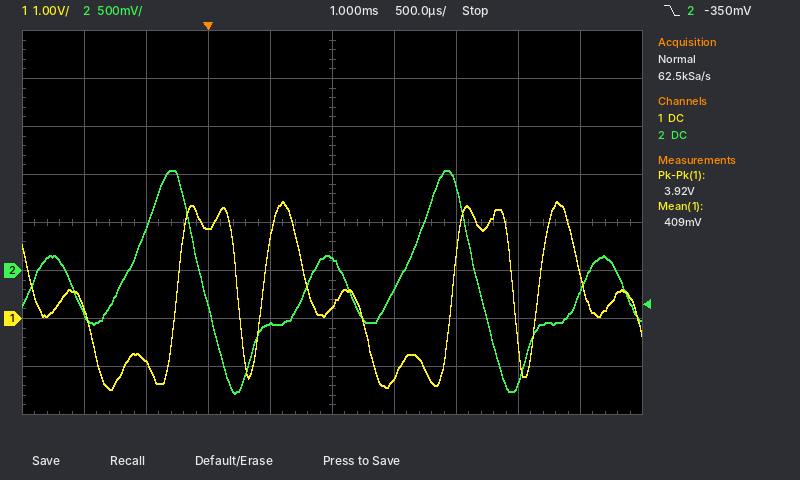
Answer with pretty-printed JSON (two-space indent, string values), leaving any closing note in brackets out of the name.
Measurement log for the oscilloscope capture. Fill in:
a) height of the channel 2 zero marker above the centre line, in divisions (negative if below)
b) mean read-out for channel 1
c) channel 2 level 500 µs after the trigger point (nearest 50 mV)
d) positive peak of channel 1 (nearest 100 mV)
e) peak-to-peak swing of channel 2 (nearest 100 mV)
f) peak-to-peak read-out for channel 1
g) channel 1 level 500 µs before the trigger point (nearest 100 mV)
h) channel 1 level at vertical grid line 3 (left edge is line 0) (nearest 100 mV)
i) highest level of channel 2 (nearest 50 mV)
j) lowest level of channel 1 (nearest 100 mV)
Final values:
{
  "height of the channel 2 zero marker above the centre line, in divisions": "-1.0 div",
  "mean read-out for channel 1": "409 mV",
  "channel 2 level 500 µs after the trigger point": "-550 mV",
  "positive peak of channel 1": "2.4 V",
  "peak-to-peak swing of channel 2": "2.30 V",
  "peak-to-peak read-out for channel 1": "3.92 V",
  "channel 1 level 500 µs before the trigger point": "-900 mV",
  "channel 1 level at vertical grid line 3 (left edge is line 0)": "1.9 V",
  "highest level of channel 2": "1.05 V",
  "lowest level of channel 1": "-1.5 V"
}
